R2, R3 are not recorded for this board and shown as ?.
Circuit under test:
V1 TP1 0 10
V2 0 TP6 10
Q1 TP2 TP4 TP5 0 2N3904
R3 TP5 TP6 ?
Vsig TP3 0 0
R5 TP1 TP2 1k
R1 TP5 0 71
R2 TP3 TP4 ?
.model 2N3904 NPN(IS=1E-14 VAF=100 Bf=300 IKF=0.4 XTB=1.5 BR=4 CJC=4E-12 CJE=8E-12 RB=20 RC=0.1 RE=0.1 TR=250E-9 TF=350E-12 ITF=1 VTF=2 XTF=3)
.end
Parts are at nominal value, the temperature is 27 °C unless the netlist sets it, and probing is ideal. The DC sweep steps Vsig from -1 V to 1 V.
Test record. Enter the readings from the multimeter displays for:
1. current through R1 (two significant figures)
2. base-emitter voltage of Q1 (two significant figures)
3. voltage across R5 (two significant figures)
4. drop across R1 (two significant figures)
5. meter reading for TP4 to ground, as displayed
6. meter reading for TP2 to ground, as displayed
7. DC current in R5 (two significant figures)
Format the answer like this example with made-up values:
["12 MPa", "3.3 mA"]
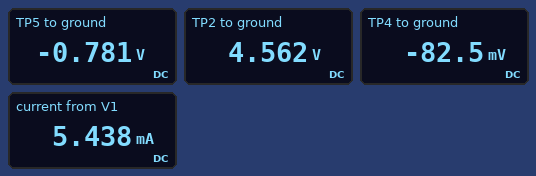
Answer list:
["11 mA", "700 mV", "5.4 V", "780 mV", "-82.5 mV", "4.562 V", "5.4 mA"]
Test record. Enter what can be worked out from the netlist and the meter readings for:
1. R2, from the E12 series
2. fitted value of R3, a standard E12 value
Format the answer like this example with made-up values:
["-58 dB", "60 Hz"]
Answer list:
["4.7 kΩ", "560 Ω"]
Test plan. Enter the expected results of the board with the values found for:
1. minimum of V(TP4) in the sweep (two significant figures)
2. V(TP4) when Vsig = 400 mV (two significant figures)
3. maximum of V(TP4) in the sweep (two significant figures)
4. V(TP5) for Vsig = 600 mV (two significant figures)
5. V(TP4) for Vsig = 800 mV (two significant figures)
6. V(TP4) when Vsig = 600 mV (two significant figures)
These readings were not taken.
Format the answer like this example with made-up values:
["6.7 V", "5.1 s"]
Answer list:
["-1.0 V", "240 mV", "260 mV", "-470 mV", "260 mV", "250 mV"]
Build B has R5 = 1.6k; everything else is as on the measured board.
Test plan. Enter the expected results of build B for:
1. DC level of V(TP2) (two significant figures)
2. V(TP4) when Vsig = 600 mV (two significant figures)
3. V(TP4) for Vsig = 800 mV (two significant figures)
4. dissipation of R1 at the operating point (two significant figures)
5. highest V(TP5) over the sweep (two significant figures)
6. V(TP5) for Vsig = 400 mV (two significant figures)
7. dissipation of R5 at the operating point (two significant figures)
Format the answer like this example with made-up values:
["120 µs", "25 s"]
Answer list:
["1.4 V", "11 mV", "15 mV", "8.7 mW", "-690 mV", "-700 mV", "47 mW"]
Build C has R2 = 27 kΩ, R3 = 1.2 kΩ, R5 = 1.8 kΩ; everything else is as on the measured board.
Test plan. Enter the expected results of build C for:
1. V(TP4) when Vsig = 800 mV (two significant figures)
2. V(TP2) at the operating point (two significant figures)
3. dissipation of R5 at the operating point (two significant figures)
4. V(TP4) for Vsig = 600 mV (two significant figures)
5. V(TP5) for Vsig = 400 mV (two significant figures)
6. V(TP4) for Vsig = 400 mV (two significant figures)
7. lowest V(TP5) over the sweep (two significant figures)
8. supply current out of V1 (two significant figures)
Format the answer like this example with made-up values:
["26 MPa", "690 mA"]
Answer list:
["420 mV", "10 V", "960 nW", "330 mV", "-430 mV", "240 mV", "-560 mV", "23 µA"]
